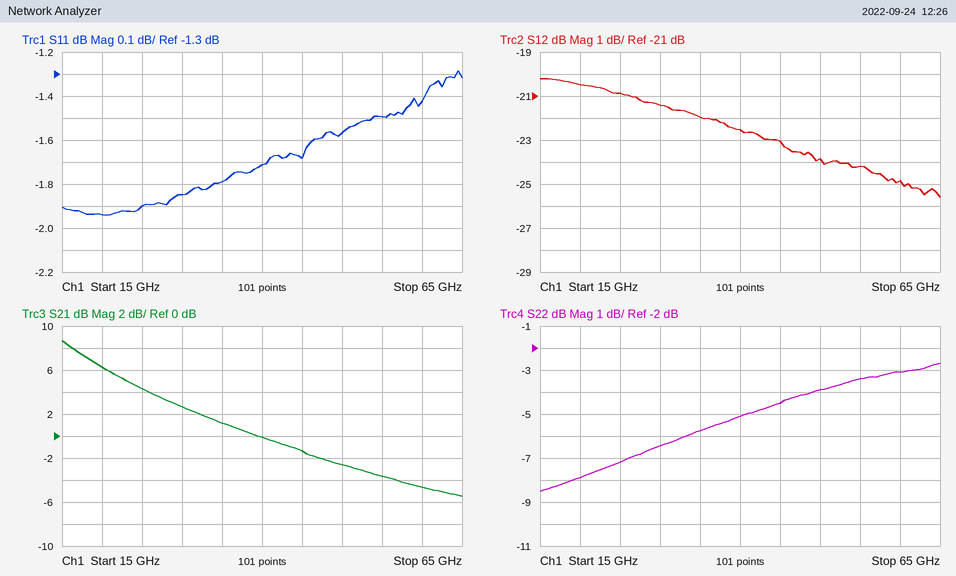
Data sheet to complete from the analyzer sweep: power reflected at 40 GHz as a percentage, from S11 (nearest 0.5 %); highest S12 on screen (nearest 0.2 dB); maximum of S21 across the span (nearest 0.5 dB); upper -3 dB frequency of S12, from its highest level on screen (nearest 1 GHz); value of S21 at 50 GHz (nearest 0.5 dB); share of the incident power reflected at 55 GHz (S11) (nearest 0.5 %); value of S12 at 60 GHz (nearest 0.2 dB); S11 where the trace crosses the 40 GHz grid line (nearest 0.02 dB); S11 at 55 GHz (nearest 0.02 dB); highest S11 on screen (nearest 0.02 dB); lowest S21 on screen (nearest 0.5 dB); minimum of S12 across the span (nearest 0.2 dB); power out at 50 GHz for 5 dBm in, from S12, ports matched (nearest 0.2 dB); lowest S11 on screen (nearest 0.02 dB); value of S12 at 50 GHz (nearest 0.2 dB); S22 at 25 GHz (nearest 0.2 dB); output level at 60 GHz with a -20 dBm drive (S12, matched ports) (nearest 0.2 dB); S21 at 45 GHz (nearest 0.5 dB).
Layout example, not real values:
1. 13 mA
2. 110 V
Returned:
1. 67.5 %
2. -20.2 dB
3. 8.5 dB
4. 45 GHz
5. -2.5 dB
6. 71.0 %
7. -24.8 dB
8. -1.72 dB
9. -1.50 dB
10. -1.28 dB
11. -5.5 dB
12. -25.6 dB
13. -18.8 dBm
14. -1.94 dB
15. -23.8 dB
16. -7.2 dB
17. -44.8 dBm
18. -1.5 dB
